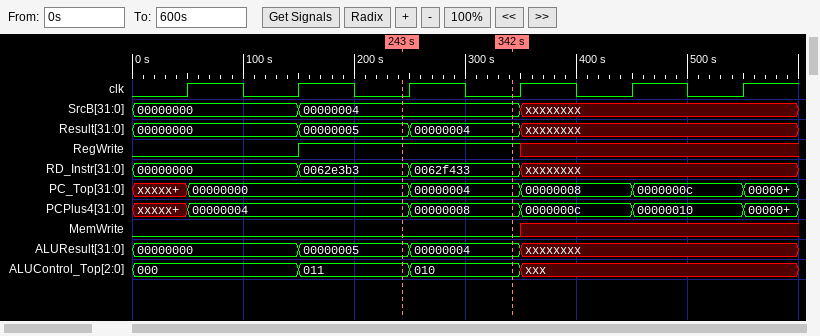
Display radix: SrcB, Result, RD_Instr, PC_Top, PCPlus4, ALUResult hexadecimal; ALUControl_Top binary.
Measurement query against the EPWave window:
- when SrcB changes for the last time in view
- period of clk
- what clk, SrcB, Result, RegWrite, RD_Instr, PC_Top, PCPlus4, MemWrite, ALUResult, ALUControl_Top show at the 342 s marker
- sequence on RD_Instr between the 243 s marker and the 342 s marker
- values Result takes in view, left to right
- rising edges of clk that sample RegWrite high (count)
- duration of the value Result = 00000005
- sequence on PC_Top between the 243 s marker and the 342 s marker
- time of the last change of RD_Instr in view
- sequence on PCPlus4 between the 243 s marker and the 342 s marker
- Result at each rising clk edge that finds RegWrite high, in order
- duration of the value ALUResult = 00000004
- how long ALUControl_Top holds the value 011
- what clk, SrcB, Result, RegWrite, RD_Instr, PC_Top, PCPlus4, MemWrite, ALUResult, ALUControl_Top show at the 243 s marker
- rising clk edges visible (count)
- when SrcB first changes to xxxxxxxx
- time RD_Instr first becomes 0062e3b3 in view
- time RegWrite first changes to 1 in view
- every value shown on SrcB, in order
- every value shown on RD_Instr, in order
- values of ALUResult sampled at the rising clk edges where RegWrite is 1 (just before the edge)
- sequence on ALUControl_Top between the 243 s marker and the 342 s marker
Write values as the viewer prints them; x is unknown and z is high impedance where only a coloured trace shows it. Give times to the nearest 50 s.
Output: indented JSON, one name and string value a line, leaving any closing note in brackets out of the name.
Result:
{
  "when SrcB changes for the last time in view": "350 s",
  "period of clk": "100 s",
  "what clk, SrcB, Result, RegWrite, RD_Instr, PC_Top, PCPlus4, MemWrite, ALUResult, ALUControl_Top show at the 342 s marker": "clk=0, SrcB=00000004, Result=00000004, RegWrite=1, RD_Instr=0062f433, PC_Top=00000004, PCPlus4=00000008, MemWrite=0, ALUResult=00000004, ALUControl_Top=010",
  "sequence on RD_Instr between the 243 s marker and the 342 s marker": "0062e3b3, 0062f433",
  "values Result takes in view, left to right": "00000000, 00000005, 00000004, xxxxxxxx",
  "rising edges of clk that sample RegWrite high": "2",
  "duration of the value Result = 00000005": "100 s",
  "sequence on PC_Top between the 243 s marker and the 342 s marker": "00000000, 00000004",
  "time of the last change of RD_Instr in view": "350 s",
  "sequence on PCPlus4 between the 243 s marker and the 342 s marker": "00000004, 00000008",
  "Result at each rising clk edge that finds RegWrite high, in order": "00000005, 00000004",
  "duration of the value ALUResult = 00000004": "100 s",
  "how long ALUControl_Top holds the value 011": "100 s",
  "what clk, SrcB, Result, RegWrite, RD_Instr, PC_Top, PCPlus4, MemWrite, ALUResult, ALUControl_Top show at the 243 s marker": "clk=0, SrcB=00000004, Result=00000005, RegWrite=1, RD_Instr=0062e3b3, PC_Top=00000000, PCPlus4=00000004, MemWrite=0, ALUResult=00000005, ALUControl_Top=011",
  "rising clk edges visible": "6",
  "when SrcB first changes to xxxxxxxx": "350 s",
  "time RD_Instr first becomes 0062e3b3 in view": "150 s",
  "time RegWrite first changes to 1 in view": "150 s",
  "every value shown on SrcB, in order": "00000000, 00000004, xxxxxxxx",
  "every value shown on RD_Instr, in order": "00000000, 0062e3b3, 0062f433, xxxxxxxx",
  "values of ALUResult sampled at the rising clk edges where RegWrite is 1": "00000005, 00000004",
  "sequence on ALUControl_Top between the 243 s marker and the 342 s marker": "011, 010"
}
